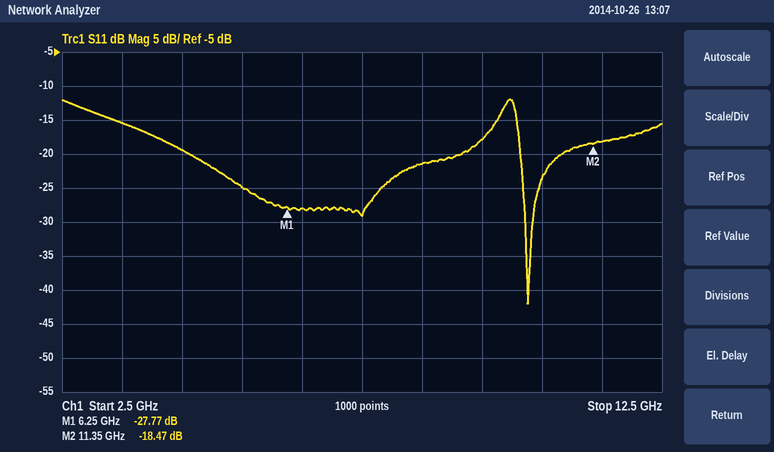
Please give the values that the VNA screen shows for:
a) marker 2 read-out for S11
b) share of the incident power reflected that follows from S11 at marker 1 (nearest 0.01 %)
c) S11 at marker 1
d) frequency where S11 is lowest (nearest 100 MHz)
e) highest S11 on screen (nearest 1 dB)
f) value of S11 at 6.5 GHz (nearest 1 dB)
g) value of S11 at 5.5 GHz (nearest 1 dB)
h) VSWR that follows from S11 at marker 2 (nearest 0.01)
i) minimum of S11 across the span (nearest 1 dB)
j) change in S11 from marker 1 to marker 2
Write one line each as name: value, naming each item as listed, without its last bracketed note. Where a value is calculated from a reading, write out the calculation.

marker 2 read-out for S11: -18.47 dB
share of the incident power reflected that follows from S11 at marker 1: 10^(-27.77/10) ≈ 0.17 %
S11 at marker 1: -27.77 dB
frequency where S11 is lowest: 10.3 GHz
highest S11 on screen: -12 dB
value of S11 at 6.5 GHz: -28 dB
value of S11 at 5.5 GHz: -25 dB
VSWR that follows from S11 at marker 2: (1 + 0.1193)/(1 − 0.1193) ≈ 1.27
minimum of S11 across the span: -42 dB
change in S11 from marker 1 to marker 2: -18.47 − (-27.77) = 9.30 dB
